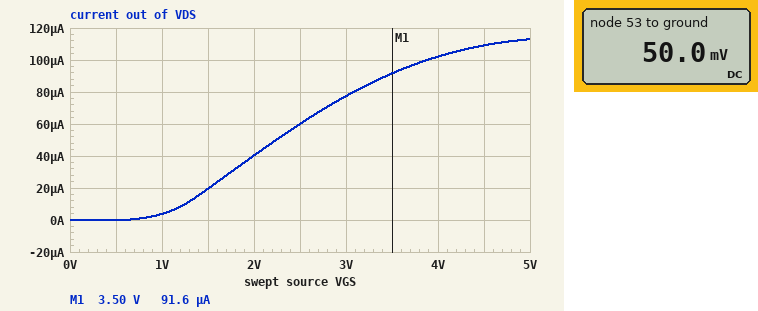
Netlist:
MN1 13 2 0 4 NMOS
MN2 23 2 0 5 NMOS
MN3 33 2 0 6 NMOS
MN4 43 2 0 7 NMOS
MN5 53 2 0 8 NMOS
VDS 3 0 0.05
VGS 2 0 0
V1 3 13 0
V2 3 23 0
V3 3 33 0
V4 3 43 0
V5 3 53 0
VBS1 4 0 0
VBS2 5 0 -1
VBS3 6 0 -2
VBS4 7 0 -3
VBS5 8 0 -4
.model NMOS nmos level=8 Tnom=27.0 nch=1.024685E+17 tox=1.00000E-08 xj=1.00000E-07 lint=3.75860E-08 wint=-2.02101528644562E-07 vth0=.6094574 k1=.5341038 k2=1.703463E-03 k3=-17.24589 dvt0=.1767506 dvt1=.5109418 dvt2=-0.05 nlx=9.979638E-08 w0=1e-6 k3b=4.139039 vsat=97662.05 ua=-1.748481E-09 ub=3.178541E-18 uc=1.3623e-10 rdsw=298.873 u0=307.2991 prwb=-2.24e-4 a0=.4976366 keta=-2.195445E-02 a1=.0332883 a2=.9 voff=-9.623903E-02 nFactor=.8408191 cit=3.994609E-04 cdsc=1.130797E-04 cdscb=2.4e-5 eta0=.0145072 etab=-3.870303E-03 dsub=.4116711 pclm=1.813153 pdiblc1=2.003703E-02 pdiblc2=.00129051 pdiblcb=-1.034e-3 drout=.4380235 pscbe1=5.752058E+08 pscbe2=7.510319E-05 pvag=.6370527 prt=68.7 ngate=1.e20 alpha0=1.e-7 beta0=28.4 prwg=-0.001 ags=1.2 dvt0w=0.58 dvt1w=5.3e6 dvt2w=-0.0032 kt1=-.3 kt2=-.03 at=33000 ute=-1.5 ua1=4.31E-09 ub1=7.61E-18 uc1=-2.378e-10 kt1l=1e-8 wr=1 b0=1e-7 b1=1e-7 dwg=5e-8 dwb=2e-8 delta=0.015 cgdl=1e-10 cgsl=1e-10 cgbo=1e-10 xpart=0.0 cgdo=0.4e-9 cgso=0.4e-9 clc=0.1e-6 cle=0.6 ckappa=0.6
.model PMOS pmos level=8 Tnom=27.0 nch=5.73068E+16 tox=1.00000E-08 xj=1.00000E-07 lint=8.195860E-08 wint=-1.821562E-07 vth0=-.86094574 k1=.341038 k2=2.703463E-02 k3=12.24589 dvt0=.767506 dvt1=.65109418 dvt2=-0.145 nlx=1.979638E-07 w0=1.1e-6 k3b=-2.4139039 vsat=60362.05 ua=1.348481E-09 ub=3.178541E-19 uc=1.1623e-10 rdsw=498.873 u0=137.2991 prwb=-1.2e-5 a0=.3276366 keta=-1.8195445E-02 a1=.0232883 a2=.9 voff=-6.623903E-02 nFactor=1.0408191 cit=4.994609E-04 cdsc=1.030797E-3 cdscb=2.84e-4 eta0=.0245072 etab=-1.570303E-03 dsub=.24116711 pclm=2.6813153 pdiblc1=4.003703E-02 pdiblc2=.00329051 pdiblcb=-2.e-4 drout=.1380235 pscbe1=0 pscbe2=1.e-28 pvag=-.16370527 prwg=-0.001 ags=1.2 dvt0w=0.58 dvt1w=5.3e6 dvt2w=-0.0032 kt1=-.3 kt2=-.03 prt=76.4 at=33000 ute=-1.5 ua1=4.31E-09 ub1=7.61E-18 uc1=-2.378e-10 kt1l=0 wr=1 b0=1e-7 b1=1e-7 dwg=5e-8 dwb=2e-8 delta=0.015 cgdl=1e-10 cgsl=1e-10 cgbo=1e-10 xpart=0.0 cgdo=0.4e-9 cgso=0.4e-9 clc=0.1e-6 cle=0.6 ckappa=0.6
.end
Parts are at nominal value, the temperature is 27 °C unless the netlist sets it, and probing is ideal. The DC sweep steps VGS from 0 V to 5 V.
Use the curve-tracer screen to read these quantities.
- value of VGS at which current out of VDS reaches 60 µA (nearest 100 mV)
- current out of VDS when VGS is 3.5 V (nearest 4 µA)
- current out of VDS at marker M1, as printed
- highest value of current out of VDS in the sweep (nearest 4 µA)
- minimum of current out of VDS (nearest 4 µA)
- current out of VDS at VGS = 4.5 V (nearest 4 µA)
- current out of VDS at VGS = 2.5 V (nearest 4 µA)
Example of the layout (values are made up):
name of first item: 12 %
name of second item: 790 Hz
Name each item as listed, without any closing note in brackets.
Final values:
value of VGS at which current out of VDS reaches 60 µA: 2.5 V
current out of VDS when VGS is 3.5 V: 92 µA
current out of VDS at marker M1, as printed: 91.6 µA
highest value of current out of VDS in the sweep: 112 µA
minimum of current out of VDS: 0 A
current out of VDS at VGS = 4.5 V: 108 µA
current out of VDS at VGS = 2.5 V: 60 µA
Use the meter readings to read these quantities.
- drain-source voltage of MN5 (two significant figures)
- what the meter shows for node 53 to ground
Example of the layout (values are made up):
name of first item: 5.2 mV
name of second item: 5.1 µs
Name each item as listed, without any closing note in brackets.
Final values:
drain-source voltage of MN5: 50 mV
what the meter shows for node 53 to ground: 50.0 mV
